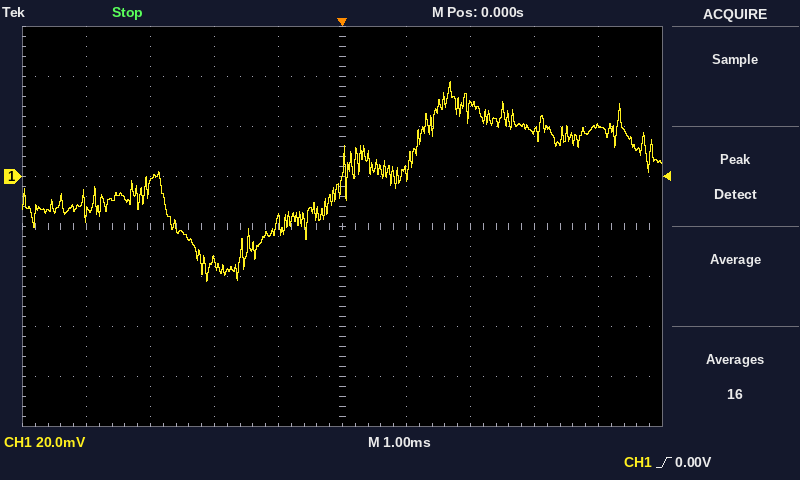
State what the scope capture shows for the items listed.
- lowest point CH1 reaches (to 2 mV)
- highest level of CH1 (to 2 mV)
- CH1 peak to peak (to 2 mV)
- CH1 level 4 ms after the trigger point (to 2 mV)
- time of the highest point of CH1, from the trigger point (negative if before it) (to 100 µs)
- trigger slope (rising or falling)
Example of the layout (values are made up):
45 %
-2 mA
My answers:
-42 mV
38 mV
80 mV
20 mV
+1.7 ms
rising
